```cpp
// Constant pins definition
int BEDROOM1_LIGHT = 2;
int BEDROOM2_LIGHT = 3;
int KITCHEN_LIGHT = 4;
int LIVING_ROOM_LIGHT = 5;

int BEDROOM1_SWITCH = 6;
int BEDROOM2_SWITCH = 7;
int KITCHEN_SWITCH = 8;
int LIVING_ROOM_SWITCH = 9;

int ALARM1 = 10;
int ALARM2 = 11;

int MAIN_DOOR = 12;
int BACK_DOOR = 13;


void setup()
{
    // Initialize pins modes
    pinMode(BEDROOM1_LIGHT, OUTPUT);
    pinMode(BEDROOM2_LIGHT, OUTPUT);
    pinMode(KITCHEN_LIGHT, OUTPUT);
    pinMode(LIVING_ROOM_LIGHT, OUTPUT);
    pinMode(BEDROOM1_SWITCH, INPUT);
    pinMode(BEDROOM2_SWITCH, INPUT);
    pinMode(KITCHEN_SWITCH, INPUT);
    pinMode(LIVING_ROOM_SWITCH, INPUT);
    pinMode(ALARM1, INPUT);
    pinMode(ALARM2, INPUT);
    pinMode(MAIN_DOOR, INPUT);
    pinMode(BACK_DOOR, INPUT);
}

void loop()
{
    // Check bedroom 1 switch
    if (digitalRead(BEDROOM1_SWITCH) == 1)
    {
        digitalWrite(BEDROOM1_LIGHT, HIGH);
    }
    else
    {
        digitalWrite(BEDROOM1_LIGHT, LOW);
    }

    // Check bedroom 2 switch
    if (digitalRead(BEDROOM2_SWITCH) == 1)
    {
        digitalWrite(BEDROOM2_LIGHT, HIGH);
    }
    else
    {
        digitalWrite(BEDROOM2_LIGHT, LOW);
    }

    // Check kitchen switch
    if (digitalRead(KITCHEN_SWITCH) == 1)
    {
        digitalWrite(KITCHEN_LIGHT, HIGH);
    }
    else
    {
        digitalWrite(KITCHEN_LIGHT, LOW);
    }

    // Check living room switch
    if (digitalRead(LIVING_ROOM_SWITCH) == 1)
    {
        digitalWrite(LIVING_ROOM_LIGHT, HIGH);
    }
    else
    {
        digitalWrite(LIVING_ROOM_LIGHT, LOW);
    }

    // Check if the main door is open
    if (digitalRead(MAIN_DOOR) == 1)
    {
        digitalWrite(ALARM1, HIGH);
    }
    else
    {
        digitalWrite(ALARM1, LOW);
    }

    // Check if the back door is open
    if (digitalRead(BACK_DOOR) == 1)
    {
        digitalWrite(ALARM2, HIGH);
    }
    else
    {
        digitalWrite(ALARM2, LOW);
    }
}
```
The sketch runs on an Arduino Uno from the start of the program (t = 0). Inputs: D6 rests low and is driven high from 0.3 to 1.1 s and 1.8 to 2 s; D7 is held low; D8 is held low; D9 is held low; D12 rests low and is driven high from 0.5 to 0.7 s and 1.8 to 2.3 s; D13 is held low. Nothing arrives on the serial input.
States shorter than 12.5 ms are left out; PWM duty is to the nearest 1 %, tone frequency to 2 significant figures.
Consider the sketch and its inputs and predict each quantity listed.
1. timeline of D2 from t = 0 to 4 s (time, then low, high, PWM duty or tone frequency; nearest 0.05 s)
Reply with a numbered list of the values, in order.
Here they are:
1. 0 s low; 0.3 s high; 1.1 s low; 1.8 s high; 2 s low
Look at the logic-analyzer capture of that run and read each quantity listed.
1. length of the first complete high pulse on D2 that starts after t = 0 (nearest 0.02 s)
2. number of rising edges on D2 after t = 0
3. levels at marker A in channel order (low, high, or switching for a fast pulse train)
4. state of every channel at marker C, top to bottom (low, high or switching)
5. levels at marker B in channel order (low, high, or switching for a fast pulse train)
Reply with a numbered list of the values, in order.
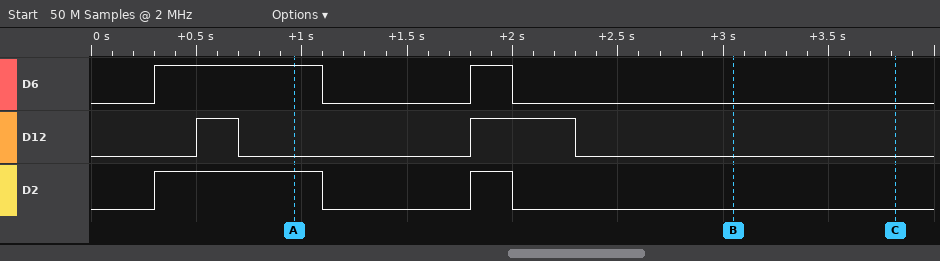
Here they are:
1. 0.80 s
2. 2
3. D6 high, D12 low, D2 high
4. D6 low, D12 low, D2 low
5. D6 low, D12 low, D2 low
